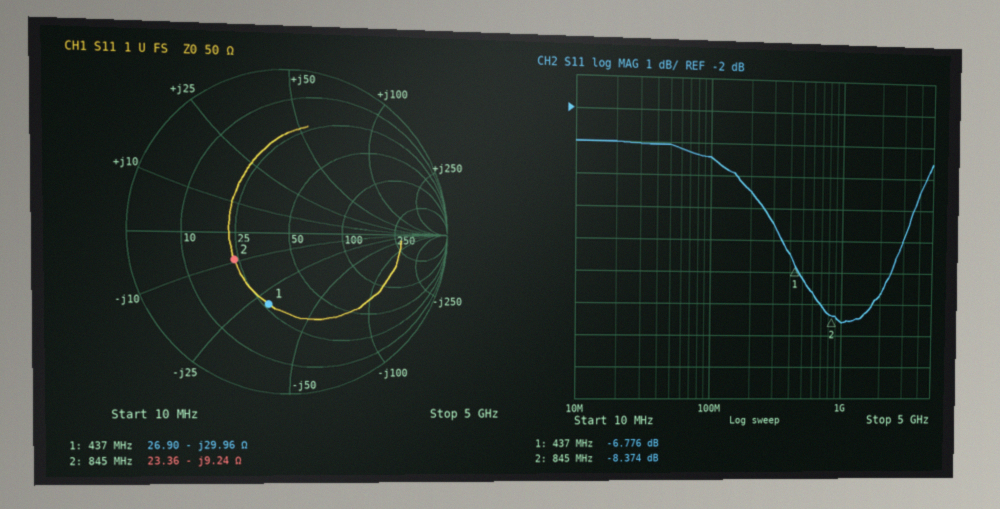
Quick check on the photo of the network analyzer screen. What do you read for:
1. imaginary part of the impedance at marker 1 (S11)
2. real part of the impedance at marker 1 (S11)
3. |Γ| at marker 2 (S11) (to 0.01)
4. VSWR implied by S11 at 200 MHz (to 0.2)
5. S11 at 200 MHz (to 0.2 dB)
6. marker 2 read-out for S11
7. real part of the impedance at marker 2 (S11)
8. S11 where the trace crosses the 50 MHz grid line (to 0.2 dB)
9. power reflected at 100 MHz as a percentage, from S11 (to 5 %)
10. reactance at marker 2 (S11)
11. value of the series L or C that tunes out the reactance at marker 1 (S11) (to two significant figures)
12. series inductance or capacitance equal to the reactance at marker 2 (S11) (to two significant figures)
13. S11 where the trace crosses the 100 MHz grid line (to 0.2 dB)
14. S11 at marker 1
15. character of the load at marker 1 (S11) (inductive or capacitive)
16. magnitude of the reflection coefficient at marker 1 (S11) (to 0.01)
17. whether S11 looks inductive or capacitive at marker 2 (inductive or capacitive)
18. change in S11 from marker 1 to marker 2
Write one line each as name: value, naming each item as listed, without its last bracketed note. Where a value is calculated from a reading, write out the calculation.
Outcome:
imaginary part of the impedance at marker 1: -29.96 Ω
real part of the impedance at marker 1: 26.90 Ω
|Γ| at marker 2 (S11): 0.38
VSWR implied by S11 at 200 MHz: |Γ| = 10^(-4.4/20) = 0.6026; VSWR = (1 + 0.6026)/(1 − 0.6026) ≈ 4.0
S11 at 200 MHz: -4.4 dB
marker 2 read-out for S11: -8.374 dB
real part of the impedance at marker 2: 23.36 Ω
S11 where the trace crosses the 50 MHz grid line: -3.0 dB
power reflected at 100 MHz as a percentage, from S11: 10^(-3.4/10) ≈ 45.7 %, so 45 % to the nearest 5 %
reactance at marker 2: -9.24 Ω
value of the series L or C that tunes out the reactance at marker 1 (S11): L = 29.96 Ω/(2π × 437 MHz) ≈ 11 nH
series inductance or capacitance equal to the reactance at marker 2 (S11): C = 1/(2π × 845 MHz × 9.24 Ω) ≈ 20 pF
S11 where the trace crosses the 100 MHz grid line: -3.4 dB
S11 at marker 1: -6.776 dB
character of the load at marker 1 (S11): capacitive
magnitude of the reflection coefficient at marker 1 (S11): 0.46
whether S11 looks inductive or capacitive at marker 2: capacitive
change in S11 from marker 1 to marker 2: -8.374 − (-6.776) = -1.598 dB
